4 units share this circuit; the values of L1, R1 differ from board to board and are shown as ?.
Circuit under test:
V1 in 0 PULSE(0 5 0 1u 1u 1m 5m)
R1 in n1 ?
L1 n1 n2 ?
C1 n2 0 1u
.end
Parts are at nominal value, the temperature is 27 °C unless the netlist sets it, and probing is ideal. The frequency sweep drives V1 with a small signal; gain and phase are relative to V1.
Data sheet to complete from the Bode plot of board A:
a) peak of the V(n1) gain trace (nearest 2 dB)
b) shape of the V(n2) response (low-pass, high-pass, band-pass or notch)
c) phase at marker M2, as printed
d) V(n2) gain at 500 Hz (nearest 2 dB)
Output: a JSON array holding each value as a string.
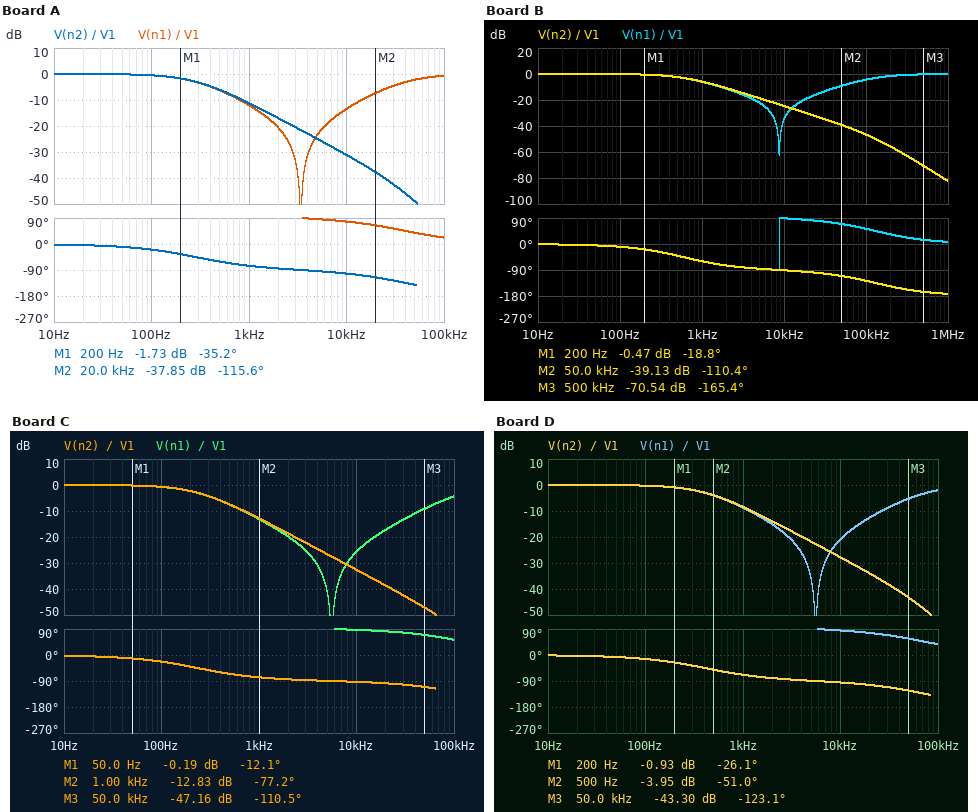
["0 dB", "low-pass", "-115.6 deg", "-6 dB"]
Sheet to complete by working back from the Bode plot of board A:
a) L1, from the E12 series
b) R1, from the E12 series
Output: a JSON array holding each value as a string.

["2.2 mH", "560 Ω"]
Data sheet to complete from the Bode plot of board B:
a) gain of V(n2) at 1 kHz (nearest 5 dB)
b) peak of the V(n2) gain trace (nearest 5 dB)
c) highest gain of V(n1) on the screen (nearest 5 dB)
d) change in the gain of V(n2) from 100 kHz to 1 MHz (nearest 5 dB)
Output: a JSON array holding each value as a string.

["-5 dB", "0 dB", "0 dB", "-35 dB"]
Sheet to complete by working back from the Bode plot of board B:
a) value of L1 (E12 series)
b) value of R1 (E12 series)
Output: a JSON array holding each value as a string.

["330 µH", "270 Ω"]
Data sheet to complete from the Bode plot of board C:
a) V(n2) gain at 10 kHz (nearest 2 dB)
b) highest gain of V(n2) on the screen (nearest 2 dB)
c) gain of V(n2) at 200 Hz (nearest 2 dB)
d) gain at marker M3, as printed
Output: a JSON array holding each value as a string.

["-32 dB", "0 dB", "-2 dB", "-47.16 dB"]
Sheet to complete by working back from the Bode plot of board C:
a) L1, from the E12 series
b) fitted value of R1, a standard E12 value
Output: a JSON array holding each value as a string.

["820 µH", "680 Ω"]
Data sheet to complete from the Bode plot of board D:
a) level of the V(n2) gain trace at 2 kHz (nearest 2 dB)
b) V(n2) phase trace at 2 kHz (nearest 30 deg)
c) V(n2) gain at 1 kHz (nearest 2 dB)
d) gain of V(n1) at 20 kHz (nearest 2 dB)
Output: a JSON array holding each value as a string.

["-14 dB", "-90 deg", "-8 dB", "-12 dB"]
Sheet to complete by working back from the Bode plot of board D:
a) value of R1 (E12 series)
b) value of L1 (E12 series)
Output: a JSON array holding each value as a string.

["390 Ω", "820 µH"]
